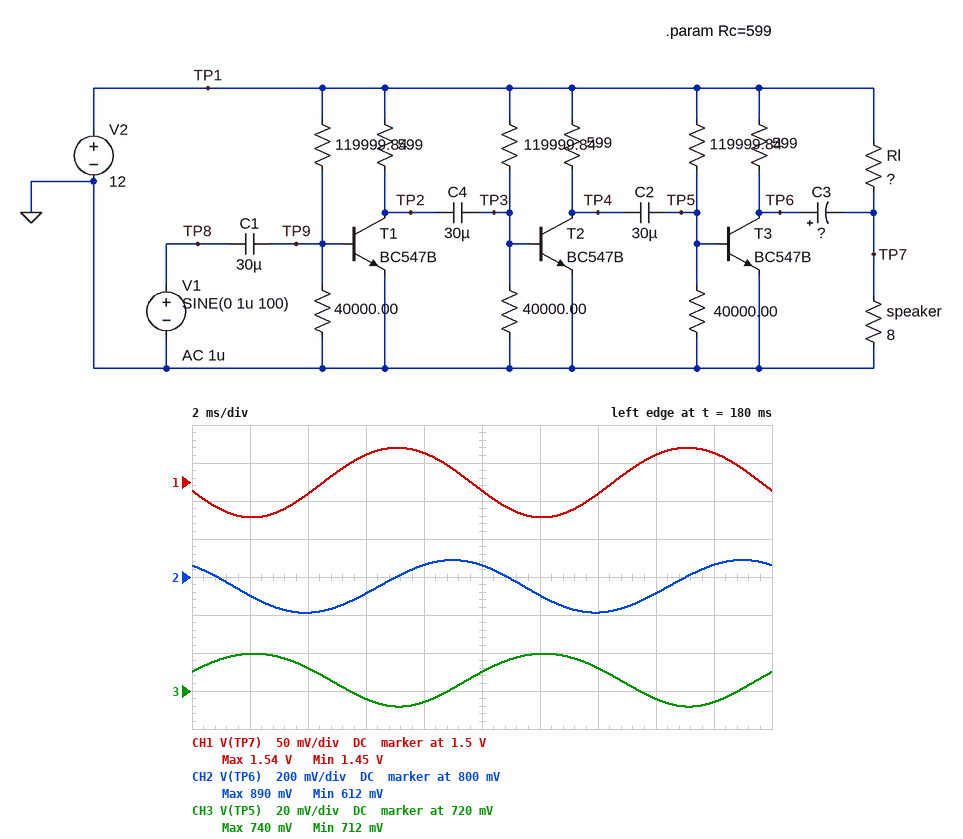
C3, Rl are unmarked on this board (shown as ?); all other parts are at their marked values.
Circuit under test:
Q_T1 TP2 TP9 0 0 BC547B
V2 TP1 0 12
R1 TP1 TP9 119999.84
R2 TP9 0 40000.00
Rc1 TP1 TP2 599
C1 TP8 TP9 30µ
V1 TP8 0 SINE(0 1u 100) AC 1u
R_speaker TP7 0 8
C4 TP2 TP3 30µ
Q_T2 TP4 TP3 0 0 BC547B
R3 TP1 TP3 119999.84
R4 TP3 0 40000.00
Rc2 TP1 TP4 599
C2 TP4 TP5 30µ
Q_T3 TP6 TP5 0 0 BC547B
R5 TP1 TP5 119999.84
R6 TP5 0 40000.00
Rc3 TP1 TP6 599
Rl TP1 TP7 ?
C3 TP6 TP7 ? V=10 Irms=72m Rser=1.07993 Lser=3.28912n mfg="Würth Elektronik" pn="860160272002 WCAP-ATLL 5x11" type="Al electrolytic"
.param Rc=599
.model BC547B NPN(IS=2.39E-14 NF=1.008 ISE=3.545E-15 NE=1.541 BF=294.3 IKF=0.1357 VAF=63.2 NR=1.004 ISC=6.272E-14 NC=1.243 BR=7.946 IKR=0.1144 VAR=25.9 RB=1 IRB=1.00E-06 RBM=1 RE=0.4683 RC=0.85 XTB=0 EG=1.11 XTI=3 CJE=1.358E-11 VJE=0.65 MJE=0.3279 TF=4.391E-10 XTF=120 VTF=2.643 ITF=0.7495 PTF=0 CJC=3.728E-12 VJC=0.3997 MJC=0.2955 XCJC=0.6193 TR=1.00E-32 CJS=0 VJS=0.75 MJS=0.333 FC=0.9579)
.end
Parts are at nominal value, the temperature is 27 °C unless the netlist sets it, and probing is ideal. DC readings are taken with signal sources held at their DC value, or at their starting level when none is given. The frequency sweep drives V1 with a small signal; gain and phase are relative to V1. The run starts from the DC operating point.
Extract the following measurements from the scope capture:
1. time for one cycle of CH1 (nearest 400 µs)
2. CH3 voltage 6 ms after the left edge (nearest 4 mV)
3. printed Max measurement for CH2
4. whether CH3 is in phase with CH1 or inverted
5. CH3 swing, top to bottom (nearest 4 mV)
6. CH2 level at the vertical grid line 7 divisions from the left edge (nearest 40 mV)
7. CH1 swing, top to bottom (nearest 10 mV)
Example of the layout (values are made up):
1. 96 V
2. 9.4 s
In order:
1. 10.0 ms
2. 716 mV
3. 890 mV
4. inverted
5. 28 mV
6. 600 mV
7. 90 mV
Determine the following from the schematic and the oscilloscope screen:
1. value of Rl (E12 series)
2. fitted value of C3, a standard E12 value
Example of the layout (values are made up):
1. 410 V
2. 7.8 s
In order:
1. 56 Ω
2. 82 µF
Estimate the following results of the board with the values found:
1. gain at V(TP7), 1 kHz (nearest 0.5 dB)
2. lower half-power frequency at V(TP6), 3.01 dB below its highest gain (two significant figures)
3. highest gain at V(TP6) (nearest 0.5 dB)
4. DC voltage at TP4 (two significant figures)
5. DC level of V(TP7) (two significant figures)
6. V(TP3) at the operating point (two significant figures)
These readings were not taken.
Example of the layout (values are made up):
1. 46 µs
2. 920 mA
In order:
1. 93.5 dB
2. 5.8 Hz
3. 115.5 dB
4. 690 mV
5. 1.5 V
6. 730 mV
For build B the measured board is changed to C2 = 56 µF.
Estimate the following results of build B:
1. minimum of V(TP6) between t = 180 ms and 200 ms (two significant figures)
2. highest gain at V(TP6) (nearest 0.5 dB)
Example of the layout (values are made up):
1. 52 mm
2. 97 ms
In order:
1. 600 mV
2. 116.5 dB
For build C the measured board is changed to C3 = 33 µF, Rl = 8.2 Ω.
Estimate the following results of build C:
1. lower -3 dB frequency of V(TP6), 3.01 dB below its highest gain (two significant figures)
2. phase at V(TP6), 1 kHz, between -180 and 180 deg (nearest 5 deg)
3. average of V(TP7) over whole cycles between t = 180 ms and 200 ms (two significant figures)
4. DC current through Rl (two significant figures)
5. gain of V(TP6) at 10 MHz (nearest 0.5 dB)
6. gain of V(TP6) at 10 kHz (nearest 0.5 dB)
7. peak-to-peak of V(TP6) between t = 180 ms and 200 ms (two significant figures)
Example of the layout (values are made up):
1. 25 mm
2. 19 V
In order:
1. 7.3 Hz
2. 140 deg
3. 5.9 V
4. 740 mA
5. 60.0 dB
6. 91.0 dB
7. 640 mV
